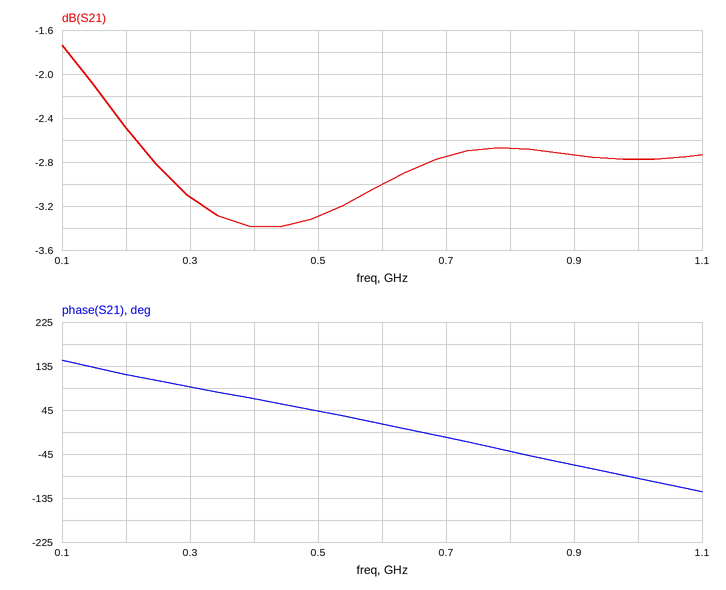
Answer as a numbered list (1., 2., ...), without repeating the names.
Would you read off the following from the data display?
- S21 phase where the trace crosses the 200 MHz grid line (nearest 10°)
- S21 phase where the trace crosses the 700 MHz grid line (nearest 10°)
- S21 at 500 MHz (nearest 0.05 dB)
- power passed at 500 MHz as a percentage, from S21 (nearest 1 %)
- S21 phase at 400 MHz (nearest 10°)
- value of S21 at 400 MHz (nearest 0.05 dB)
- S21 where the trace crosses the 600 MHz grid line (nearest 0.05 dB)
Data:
1. 120°
2. -10°
3. -3.30 dB
4. 47 %
5. 70°
6. -3.40 dB
7. -3.00 dB
